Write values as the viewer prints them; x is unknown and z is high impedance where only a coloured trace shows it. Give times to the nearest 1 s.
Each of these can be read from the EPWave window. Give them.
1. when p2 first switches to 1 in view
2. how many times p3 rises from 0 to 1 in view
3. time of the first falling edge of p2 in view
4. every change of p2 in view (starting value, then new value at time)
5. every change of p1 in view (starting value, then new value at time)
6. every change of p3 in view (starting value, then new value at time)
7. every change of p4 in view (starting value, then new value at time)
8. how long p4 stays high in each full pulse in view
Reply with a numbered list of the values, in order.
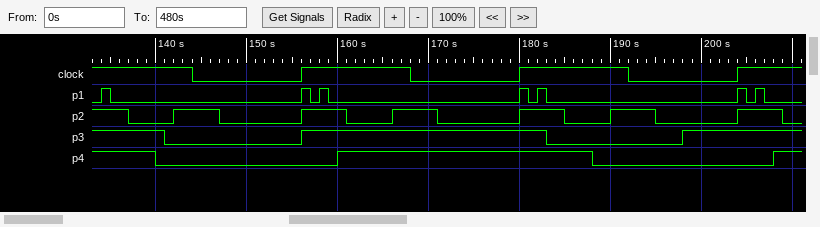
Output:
1. 142 s
2. 2
3. 137 s
4. 1, 0 at 137 s, 1 at 142 s, 0 at 147 s, 1 at 156 s, 0 at 161 s, 1 at 166 s, 0 at 171 s, 1 at 180 s, 0 at 185 s, 1 at 190 s, 0 at 195 s, 1 at 204 s, 0 at 209 s
5. 0, 1 at 134 s, 0 at 135 s, 1 at 156 s, 0 at 157 s, 1 at 158 s, 0 at 159 s, 1 at 180 s, 0 at 181 s, 1 at 182 s, 0 at 183 s, 1 at 204 s, 0 at 205 s, 1 at 206 s, 0 at 207 s
6. 1, 0 at 141 s, 1 at 156 s, 0 at 183 s, 1 at 198 s
7. 1, 0 at 140 s, 1 at 160 s, 0 at 188 s, 1 at 208 s
8. 28 s
